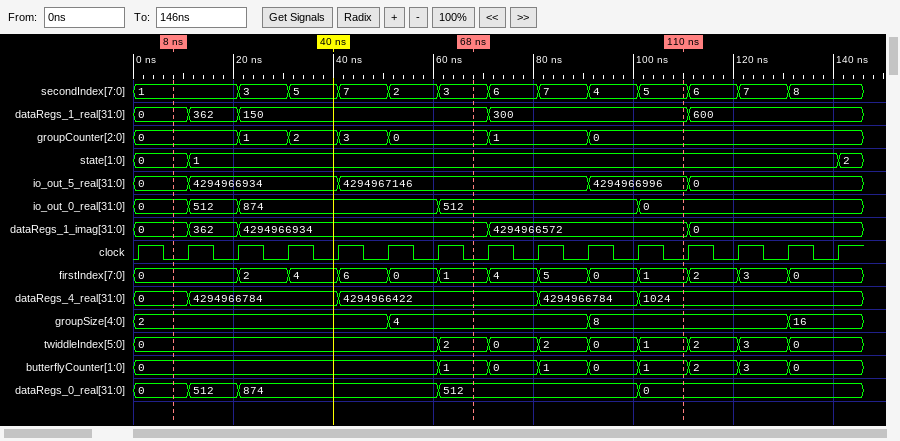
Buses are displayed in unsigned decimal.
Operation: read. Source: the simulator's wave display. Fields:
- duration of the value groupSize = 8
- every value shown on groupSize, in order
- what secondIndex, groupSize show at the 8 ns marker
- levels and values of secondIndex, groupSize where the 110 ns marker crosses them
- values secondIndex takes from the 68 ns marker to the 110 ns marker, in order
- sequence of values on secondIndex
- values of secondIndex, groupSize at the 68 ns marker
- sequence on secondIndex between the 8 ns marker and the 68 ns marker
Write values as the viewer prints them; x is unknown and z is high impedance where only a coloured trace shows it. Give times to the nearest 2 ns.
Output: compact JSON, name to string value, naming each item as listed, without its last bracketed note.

{"duration of the value groupSize = 8": "40 ns", "every value shown on groupSize, in order": "2, 4, 8, 16", "what secondIndex, groupSize show at the 8 ns marker": "secondIndex=1, groupSize=2", "levels and values of secondIndex, groupSize where the 110 ns marker crosses them": "secondIndex=5, groupSize=8", "values secondIndex takes from the 68 ns marker to the 110 ns marker, in order": "3, 6, 7, 4, 5", "sequence of values on secondIndex": "1, 3, 5, 7, 2, 3, 6, 7, 4, 5, 6, 7, 8", "values of secondIndex, groupSize at the 68 ns marker": "secondIndex=3, groupSize=4", "sequence on secondIndex between the 8 ns marker and the 68 ns marker": "1, 3, 5, 7, 2, 3"}
